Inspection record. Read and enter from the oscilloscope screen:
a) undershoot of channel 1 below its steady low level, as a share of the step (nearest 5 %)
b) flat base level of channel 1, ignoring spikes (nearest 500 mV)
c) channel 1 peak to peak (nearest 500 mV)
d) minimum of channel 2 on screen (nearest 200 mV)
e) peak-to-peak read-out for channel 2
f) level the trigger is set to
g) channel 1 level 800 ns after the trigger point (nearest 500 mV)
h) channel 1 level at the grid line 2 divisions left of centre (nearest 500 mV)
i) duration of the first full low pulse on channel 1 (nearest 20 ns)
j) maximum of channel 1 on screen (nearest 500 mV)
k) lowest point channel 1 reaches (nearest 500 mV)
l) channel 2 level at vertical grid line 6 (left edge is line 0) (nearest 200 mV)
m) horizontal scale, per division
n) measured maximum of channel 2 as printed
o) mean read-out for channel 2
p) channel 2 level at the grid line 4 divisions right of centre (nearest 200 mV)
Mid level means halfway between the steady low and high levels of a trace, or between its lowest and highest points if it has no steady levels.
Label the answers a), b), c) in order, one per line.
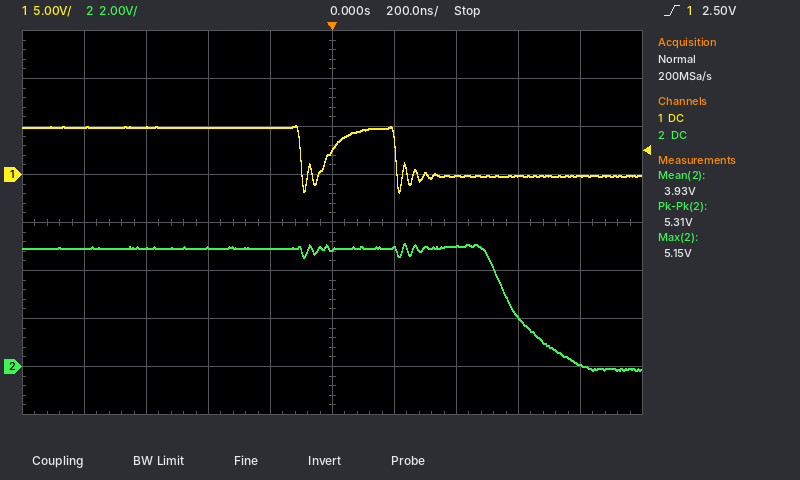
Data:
a) 35 %
b) 0.0 V
c) 7.0 V
d) -200 mV
e) 5.31 V
f) 2.50 V
g) 0.0 V
h) 5.0 V
i) 100 ns
j) 5.0 V
k) -2.0 V
l) 4.8 V
m) 200 ns
n) 5.15 V
o) 3.93 V
p) 0.0 V
